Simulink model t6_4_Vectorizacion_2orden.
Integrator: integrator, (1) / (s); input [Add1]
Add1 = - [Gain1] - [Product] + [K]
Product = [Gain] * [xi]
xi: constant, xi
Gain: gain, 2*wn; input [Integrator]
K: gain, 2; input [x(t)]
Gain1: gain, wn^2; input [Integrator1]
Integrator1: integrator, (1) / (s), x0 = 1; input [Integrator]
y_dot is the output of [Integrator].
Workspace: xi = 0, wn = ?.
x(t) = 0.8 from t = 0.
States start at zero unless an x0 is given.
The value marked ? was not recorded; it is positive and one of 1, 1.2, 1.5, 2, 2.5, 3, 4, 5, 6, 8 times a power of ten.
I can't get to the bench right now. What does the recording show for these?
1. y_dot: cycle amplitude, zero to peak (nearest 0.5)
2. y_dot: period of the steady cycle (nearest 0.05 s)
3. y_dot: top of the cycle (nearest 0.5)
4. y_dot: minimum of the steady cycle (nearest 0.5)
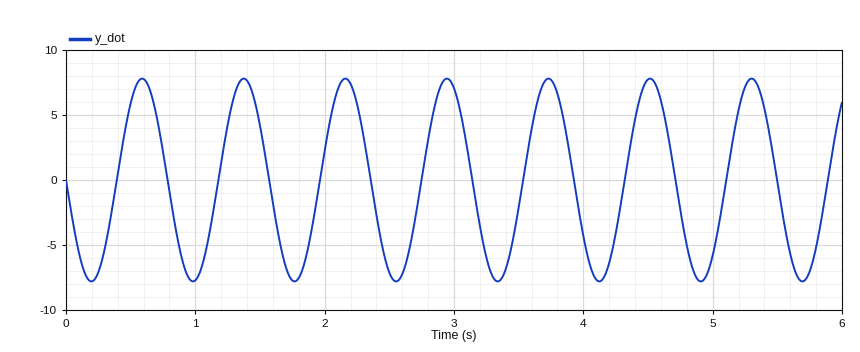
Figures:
8.0
0.80 s
8.0
-8.0
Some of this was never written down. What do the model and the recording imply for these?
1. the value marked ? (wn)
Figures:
8
